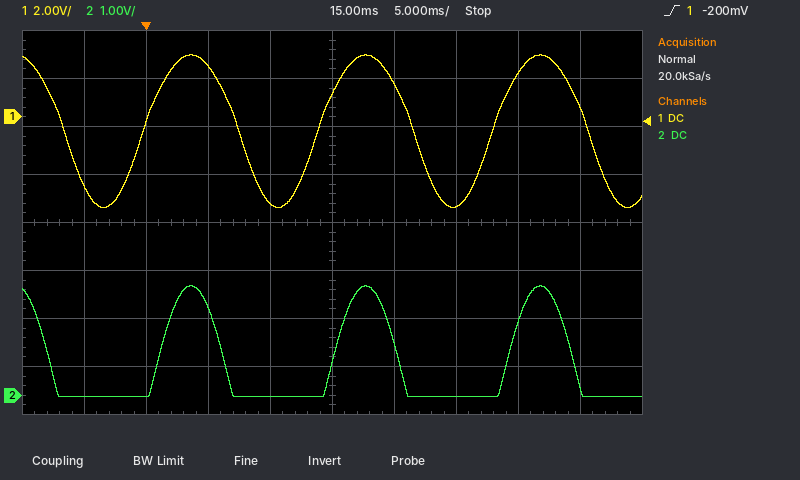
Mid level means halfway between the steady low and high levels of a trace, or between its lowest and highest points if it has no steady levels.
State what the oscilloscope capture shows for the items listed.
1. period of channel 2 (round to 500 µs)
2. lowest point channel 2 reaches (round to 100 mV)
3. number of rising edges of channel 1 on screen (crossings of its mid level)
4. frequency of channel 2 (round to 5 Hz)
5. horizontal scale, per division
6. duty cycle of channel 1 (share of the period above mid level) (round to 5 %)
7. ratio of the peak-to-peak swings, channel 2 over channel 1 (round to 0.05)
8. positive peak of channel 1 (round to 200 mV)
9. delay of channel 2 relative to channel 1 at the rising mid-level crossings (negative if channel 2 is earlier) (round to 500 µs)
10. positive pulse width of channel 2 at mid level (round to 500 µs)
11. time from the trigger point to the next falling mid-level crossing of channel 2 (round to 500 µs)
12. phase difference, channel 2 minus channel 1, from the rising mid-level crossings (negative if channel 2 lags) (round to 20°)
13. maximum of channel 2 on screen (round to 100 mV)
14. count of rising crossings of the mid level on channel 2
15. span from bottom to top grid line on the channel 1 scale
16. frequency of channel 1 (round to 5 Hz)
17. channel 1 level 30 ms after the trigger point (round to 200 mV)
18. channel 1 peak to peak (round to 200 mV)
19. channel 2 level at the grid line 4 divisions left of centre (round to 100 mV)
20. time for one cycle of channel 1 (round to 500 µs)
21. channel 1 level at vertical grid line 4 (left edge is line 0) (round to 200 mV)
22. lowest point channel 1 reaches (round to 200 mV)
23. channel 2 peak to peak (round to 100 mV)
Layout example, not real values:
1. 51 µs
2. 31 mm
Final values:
1. 14.0 ms
2. 0.0 V
3. 3
4. 70 Hz
5. 5 ms
6. 55 %
7. 0.35
8. 2.6 V
9. +1.5 ms
10. 4.5 ms
11. 6.0 ms
12. -40°
13. 2.3 V
14. 3
15. 16 V
16. 70 Hz
17. 1.8 V
18. 6.4 V
19. 0.0 V
20. 14.0 ms
21. -3.6 V
22. -3.8 V
23. 2.3 V
